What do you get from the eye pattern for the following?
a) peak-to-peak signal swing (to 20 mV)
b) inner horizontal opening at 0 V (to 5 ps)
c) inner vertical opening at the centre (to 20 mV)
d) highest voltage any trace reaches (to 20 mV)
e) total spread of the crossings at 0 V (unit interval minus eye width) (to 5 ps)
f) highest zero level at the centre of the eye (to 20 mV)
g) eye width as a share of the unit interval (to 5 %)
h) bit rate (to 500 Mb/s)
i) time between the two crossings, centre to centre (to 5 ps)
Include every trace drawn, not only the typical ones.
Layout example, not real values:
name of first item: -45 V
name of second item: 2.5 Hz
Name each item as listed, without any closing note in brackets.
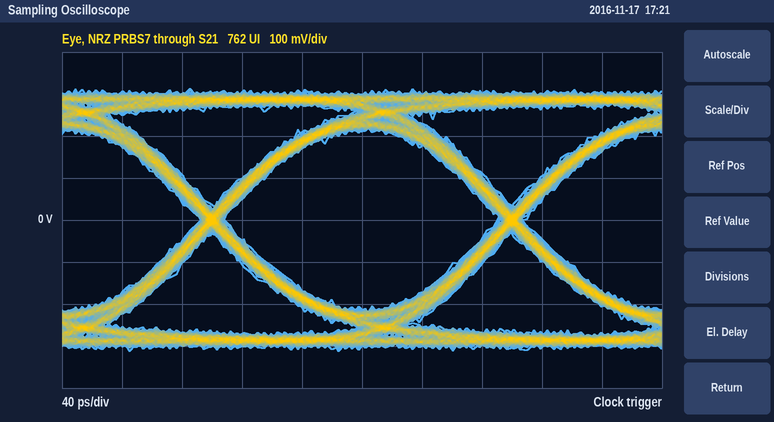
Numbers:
peak-to-peak signal swing: 620 mV
inner horizontal opening at 0 V: 180 ps
inner vertical opening at the centre: 420 mV
highest voltage any trace reaches: 320 mV
total spread of the crossings at 0 V (unit interval minus eye width): 20 ps
highest zero level at the centre of the eye: -220 mV
eye width as a share of the unit interval: 90 %
bit rate: 5.0 Gb/s
time between the two crossings, centre to centre: 200 ps
